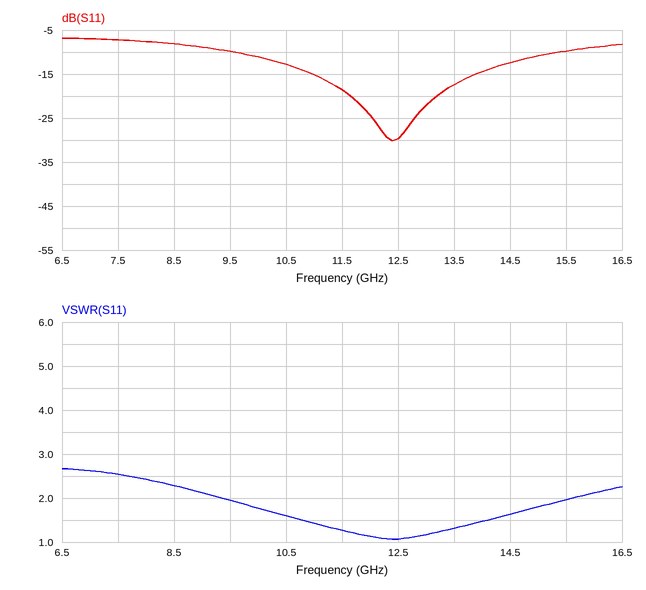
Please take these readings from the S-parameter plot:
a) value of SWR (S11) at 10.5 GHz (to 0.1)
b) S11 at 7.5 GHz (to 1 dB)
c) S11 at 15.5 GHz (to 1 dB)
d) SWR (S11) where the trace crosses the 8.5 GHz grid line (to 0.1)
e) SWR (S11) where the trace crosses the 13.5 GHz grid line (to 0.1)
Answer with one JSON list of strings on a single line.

["1.6", "-7 dB", "-10 dB", "2.3", "1.3"]
